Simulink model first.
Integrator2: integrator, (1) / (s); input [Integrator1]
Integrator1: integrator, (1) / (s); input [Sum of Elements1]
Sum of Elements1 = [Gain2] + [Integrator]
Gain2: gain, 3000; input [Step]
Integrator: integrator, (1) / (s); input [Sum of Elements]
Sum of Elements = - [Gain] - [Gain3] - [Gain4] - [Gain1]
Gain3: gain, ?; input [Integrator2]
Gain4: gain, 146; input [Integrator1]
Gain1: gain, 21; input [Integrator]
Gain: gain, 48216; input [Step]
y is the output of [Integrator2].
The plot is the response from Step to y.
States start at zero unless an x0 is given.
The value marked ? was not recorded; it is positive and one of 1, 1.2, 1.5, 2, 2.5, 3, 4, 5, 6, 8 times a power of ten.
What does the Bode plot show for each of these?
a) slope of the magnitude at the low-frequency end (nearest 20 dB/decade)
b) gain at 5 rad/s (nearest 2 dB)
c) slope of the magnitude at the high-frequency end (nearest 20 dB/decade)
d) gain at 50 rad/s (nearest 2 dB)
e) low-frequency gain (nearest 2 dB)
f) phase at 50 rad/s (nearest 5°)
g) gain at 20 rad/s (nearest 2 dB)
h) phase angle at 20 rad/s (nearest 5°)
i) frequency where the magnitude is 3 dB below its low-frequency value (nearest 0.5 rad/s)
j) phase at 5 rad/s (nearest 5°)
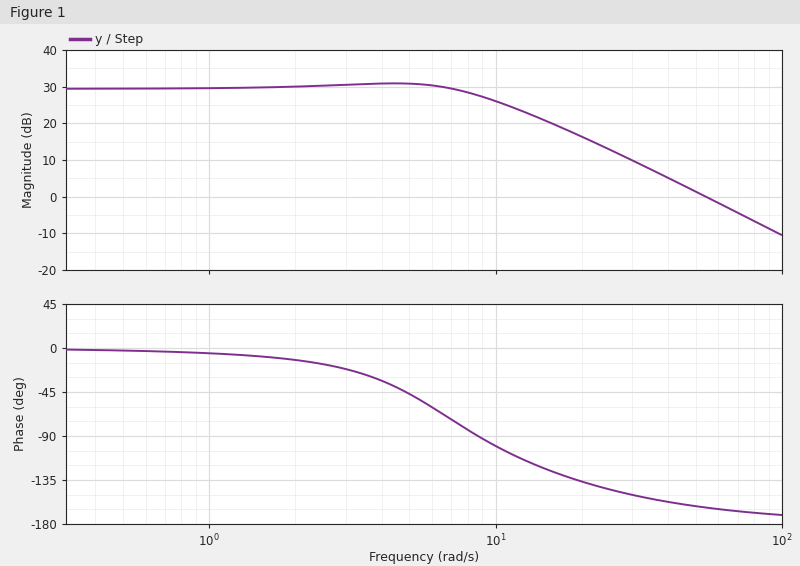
0 dB/decade
30 dB
-40 dB/decade
2 dB
30 dB
-160°
16 dB
-135°
9.5 rad/s
-45°
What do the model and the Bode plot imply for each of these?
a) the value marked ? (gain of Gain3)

500
